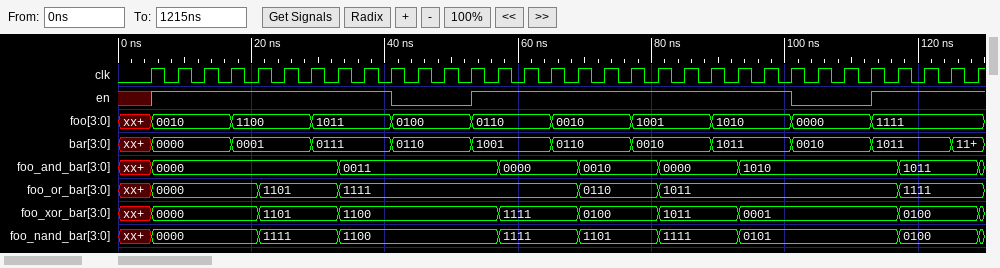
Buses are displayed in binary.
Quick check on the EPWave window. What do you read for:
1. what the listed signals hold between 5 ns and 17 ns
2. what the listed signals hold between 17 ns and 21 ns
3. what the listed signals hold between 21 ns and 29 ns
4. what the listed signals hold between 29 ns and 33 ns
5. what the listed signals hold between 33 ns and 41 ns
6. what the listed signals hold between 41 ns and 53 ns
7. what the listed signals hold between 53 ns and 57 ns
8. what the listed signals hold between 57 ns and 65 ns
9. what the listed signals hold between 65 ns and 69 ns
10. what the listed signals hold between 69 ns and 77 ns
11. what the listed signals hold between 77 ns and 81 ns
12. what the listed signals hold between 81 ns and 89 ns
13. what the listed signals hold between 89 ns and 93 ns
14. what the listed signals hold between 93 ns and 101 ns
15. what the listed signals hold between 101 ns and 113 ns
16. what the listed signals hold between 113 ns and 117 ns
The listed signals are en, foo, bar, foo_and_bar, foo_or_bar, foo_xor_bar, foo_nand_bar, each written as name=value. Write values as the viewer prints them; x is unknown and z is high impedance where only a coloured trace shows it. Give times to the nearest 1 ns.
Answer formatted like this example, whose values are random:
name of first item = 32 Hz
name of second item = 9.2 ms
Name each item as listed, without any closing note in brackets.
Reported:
what the listed signals hold between 5 ns and 17 ns = en=1, foo=0010, bar=0000, foo_and_bar=0000, foo_or_bar=0000, foo_xor_bar=0000, foo_nand_bar=0000
what the listed signals hold between 17 ns and 21 ns = en=1, foo=1100, bar=0001, foo_and_bar=0000, foo_or_bar=0000, foo_xor_bar=0000, foo_nand_bar=0000
what the listed signals hold between 21 ns and 29 ns = en=1, foo=1100, bar=0001, foo_and_bar=0000, foo_or_bar=1101, foo_xor_bar=1101, foo_nand_bar=1111
what the listed signals hold between 29 ns and 33 ns = en=1, foo=1011, bar=0111, foo_and_bar=0000, foo_or_bar=1101, foo_xor_bar=1101, foo_nand_bar=1111
what the listed signals hold between 33 ns and 41 ns = en=1, foo=1011, bar=0111, foo_and_bar=0011, foo_or_bar=1111, foo_xor_bar=1100, foo_nand_bar=1100
what the listed signals hold between 41 ns and 53 ns = en=0, foo=0100, bar=0110, foo_and_bar=0011, foo_or_bar=1111, foo_xor_bar=1100, foo_nand_bar=1100
what the listed signals hold between 53 ns and 57 ns = en=1, foo=0110, bar=1001, foo_and_bar=0011, foo_or_bar=1111, foo_xor_bar=1100, foo_nand_bar=1100
what the listed signals hold between 57 ns and 65 ns = en=1, foo=0110, bar=1001, foo_and_bar=0000, foo_or_bar=1111, foo_xor_bar=1111, foo_nand_bar=1111
what the listed signals hold between 65 ns and 69 ns = en=1, foo=0010, bar=0110, foo_and_bar=0000, foo_or_bar=1111, foo_xor_bar=1111, foo_nand_bar=1111
what the listed signals hold between 69 ns and 77 ns = en=1, foo=0010, bar=0110, foo_and_bar=0010, foo_or_bar=0110, foo_xor_bar=0100, foo_nand_bar=1101
what the listed signals hold between 77 ns and 81 ns = en=1, foo=1001, bar=0010, foo_and_bar=0010, foo_or_bar=0110, foo_xor_bar=0100, foo_nand_bar=1101
what the listed signals hold between 81 ns and 89 ns = en=1, foo=1001, bar=0010, foo_and_bar=0000, foo_or_bar=1011, foo_xor_bar=1011, foo_nand_bar=1111
what the listed signals hold between 89 ns and 93 ns = en=1, foo=1010, bar=1011, foo_and_bar=0000, foo_or_bar=1011, foo_xor_bar=1011, foo_nand_bar=1111
what the listed signals hold between 93 ns and 101 ns = en=1, foo=1010, bar=1011, foo_and_bar=1010, foo_or_bar=1011, foo_xor_bar=0001, foo_nand_bar=0101
what the listed signals hold between 101 ns and 113 ns = en=0, foo=0000, bar=0010, foo_and_bar=1010, foo_or_bar=1011, foo_xor_bar=0001, foo_nand_bar=0101
what the listed signals hold between 113 ns and 117 ns = en=1, foo=1111, bar=1011, foo_and_bar=1010, foo_or_bar=1011, foo_xor_bar=0001, foo_nand_bar=0101
